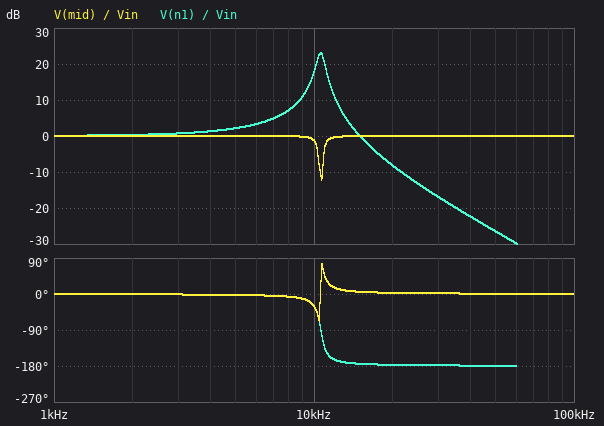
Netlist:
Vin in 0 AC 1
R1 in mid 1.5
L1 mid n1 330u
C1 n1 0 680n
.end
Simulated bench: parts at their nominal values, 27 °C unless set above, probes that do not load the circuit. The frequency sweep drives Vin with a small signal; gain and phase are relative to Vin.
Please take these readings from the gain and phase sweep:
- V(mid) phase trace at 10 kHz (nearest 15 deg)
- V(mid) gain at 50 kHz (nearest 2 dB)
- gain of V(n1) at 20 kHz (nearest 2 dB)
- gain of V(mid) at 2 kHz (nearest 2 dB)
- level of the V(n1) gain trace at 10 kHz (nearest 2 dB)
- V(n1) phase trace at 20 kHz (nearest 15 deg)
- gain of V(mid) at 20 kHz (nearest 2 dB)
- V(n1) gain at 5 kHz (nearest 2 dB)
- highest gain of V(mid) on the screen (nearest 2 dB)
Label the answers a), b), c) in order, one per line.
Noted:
a) -30 deg
b) 0 dB
c) -8 dB
d) 0 dB
e) 18 dB
f) -180 deg
g) 0 dB
h) 2 dB
i) 0 dB
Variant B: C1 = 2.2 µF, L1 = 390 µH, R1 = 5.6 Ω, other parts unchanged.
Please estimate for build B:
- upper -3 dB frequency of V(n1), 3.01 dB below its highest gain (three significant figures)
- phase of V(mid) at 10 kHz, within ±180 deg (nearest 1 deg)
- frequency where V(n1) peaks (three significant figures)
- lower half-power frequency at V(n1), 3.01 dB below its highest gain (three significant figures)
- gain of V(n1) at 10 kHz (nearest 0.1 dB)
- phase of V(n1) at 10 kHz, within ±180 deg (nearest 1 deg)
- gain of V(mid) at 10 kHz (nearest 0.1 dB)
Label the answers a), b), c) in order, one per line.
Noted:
a) 6.25 kHz
b) 18 deg
c) 5.19 kHz
d) 3.84 kHz
e) -8.0 dB
f) -162 deg
g) -0.4 dB
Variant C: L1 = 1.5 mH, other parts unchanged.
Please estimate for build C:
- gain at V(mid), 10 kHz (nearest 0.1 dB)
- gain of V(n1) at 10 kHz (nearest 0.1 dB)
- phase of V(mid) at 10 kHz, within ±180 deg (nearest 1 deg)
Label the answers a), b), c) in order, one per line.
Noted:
a) 0 dB
b) -9.6 dB
c) 1 deg
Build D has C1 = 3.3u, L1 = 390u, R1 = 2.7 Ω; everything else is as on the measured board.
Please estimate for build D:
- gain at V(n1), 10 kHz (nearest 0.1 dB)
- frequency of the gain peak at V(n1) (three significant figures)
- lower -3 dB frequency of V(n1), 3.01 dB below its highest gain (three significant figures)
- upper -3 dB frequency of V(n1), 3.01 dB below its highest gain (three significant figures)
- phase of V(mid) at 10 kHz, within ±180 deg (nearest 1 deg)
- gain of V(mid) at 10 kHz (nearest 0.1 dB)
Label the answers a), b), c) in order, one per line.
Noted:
a) -12.3 dB
b) 4.37 kHz
c) 3.77 kHz
d) 4.89 kHz
e) 8 deg
f) -0.1 dB
